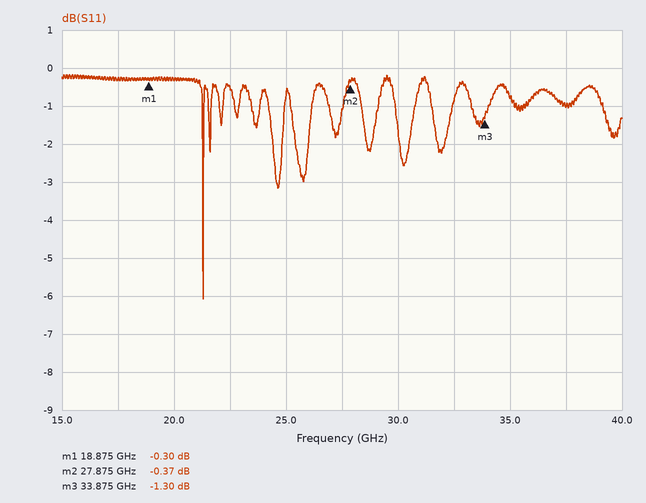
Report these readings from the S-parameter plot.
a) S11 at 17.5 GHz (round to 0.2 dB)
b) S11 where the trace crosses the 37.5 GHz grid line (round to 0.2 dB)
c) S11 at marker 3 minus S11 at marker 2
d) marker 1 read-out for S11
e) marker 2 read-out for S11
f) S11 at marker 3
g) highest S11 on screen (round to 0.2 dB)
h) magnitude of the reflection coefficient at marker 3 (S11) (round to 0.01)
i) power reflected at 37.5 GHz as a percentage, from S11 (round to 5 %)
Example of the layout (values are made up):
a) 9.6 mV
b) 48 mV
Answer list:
a) -0.2 dB
b) -1.0 dB
c) -0.93 dB
d) -0.30 dB
e) -0.37 dB
f) -1.30 dB
g) -0.2 dB
h) 0.86
i) 80 %
